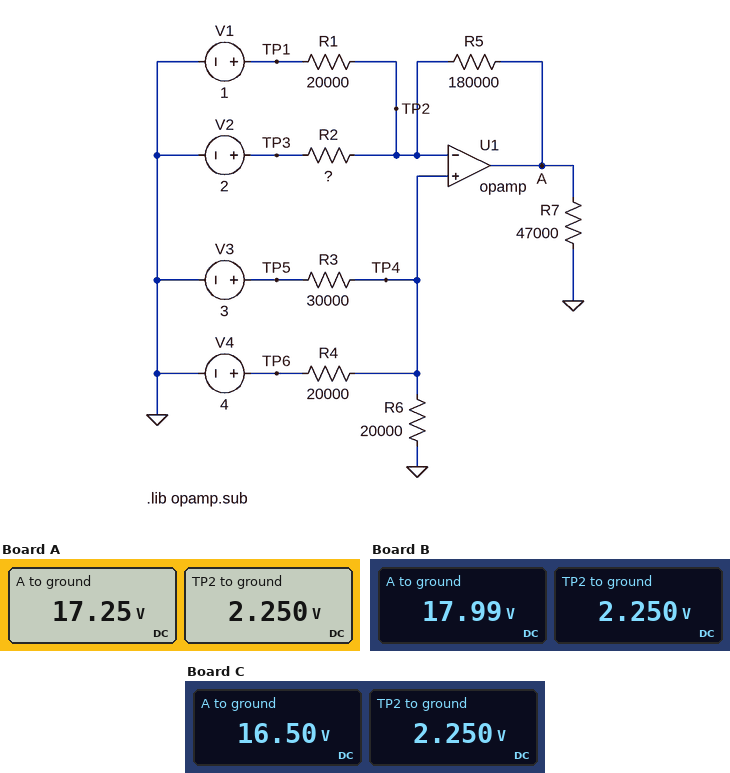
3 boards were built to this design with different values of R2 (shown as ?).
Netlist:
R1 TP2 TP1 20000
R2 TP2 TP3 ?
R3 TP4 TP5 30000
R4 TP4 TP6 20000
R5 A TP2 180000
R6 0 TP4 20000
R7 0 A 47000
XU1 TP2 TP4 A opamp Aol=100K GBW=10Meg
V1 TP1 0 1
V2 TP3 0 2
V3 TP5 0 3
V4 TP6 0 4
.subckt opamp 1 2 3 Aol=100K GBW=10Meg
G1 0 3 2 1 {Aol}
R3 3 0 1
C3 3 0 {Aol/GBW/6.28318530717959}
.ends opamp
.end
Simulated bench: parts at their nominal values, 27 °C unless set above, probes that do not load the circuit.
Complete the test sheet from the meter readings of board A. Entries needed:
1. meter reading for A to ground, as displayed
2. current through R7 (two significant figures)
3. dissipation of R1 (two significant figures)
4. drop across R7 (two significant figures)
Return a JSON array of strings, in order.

["17.25 V", "370 µA", "78 µW", "17 V"]
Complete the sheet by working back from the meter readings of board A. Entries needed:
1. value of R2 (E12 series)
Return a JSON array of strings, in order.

["12 kΩ"]
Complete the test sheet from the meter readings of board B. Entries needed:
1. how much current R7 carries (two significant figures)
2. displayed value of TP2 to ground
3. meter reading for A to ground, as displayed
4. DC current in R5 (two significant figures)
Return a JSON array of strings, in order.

["380 µA", "2.250 V", "17.99 V", "87 µA"]
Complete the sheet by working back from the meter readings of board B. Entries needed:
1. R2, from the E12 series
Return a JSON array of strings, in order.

["10 kΩ"]
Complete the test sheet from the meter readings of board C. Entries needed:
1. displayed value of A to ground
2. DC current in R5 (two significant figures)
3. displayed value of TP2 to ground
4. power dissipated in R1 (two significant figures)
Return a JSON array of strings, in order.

["16.50 V", "79 µA", "2.250 V", "78 µW"]
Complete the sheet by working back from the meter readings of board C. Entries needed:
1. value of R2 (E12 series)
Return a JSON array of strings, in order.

["15 kΩ"]
